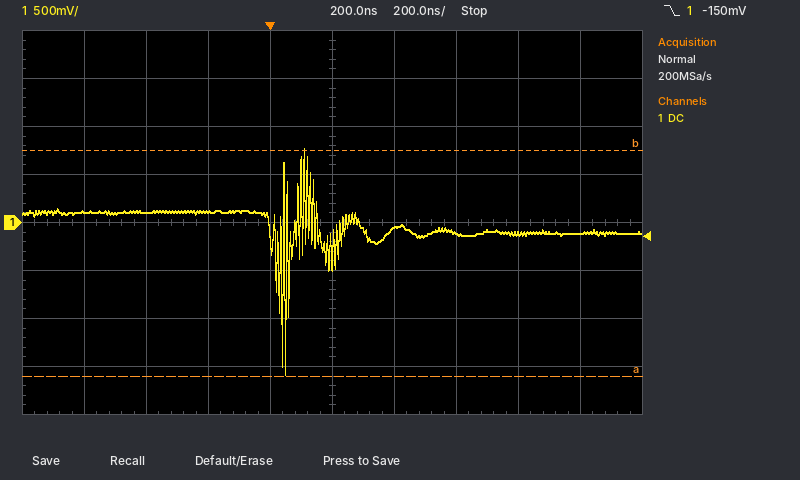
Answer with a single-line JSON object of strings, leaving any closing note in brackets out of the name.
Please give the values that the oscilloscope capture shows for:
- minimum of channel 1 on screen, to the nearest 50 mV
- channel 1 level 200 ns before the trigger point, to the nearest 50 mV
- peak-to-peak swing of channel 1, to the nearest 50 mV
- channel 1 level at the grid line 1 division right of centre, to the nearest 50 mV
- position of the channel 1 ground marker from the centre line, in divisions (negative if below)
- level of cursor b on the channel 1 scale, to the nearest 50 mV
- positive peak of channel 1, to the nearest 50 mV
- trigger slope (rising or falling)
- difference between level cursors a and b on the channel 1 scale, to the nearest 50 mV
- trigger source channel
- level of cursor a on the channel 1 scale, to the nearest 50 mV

{"minimum of channel 1 on screen, to the nearest 50 mV": "-1.60 V", "channel 1 level 200 ns before the trigger point, to the nearest 50 mV": "100 mV", "peak-to-peak swing of channel 1, to the nearest 50 mV": "2.35 V", "channel 1 level at the grid line 1 division right of centre, to the nearest 50 mV": "-50 mV", "position of the channel 1 ground marker from the centre line, in divisions": "0.0 div", "level of cursor b on the channel 1 scale, to the nearest 50 mV": "750 mV", "positive peak of channel 1, to the nearest 50 mV": "750 mV", "trigger slope": "falling", "difference between level cursors a and b on the channel 1 scale, to the nearest 50 mV": "2.35 V", "trigger source channel": "channel 1", "level of cursor a on the channel 1 scale, to the nearest 50 mV": "-1.60 V"}
